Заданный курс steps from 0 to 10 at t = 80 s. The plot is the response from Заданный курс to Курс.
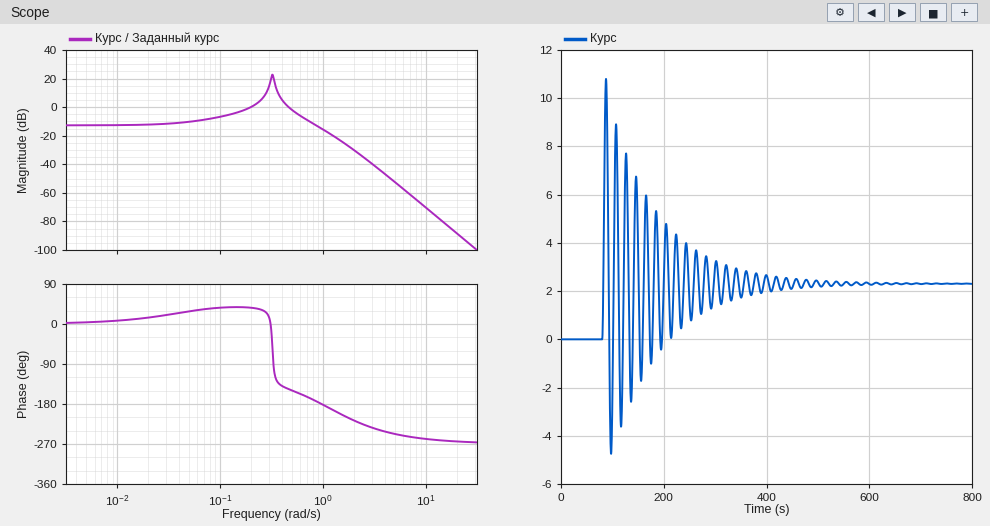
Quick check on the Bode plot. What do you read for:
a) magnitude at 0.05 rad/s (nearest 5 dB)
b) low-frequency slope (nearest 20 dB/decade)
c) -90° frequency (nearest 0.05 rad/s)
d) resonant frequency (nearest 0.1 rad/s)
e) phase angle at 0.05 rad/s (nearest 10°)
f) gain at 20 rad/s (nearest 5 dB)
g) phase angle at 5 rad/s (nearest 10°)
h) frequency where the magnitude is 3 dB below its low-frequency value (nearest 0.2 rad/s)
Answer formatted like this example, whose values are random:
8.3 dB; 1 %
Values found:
-10 dB; 0 dB/decade; 0.35 rad/s; 0.3 rad/s; 30°; -90 dB; -250°; 1.0 rad/s
